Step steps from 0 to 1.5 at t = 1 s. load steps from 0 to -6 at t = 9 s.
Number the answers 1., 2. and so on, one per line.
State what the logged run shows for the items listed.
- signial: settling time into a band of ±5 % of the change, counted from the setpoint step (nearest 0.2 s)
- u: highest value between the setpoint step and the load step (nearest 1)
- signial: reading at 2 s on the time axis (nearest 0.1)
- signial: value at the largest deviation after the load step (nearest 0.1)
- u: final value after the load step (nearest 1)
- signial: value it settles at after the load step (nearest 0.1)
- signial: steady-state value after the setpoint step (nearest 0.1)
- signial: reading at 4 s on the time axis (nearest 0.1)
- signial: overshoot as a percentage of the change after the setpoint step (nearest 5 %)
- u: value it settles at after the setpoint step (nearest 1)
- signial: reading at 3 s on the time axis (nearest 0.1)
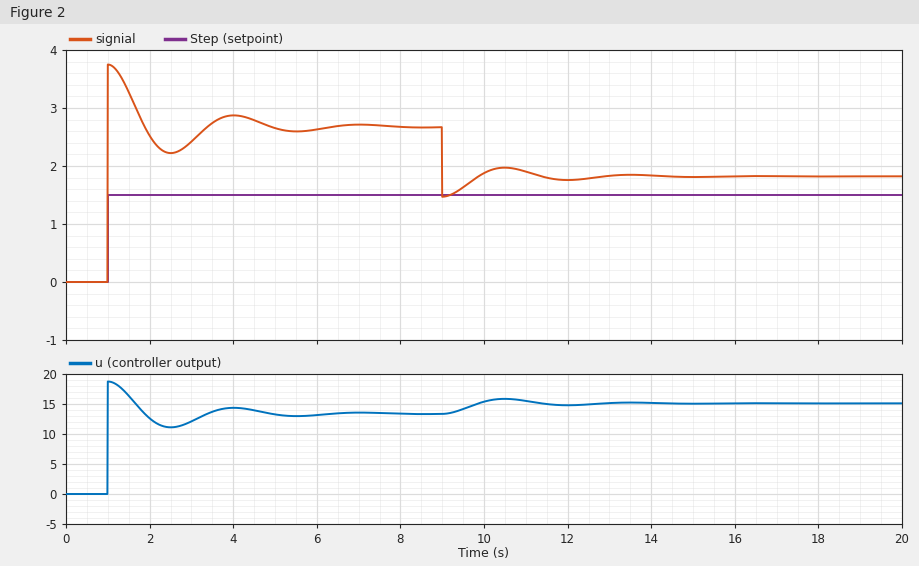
1. 3.4 s
2. 19
3. 2.5
4. 1.5
5. 15
6. 1.8
7. 2.7
8. 2.9
9. 40 %
10. 13
11. 2.4
